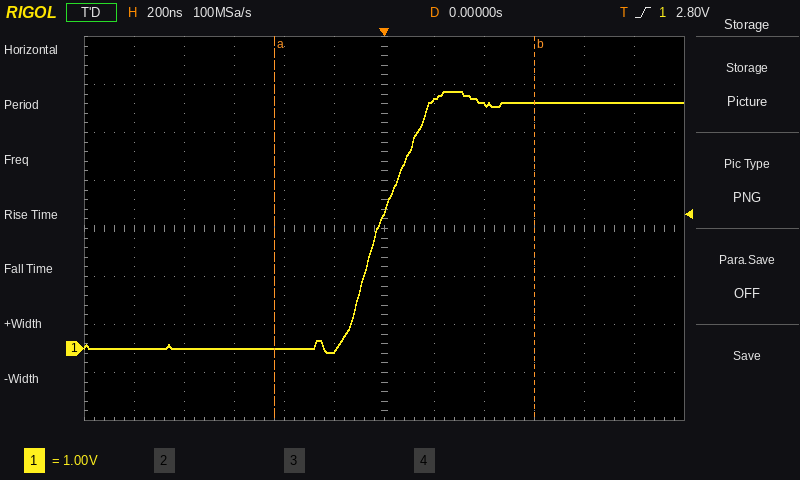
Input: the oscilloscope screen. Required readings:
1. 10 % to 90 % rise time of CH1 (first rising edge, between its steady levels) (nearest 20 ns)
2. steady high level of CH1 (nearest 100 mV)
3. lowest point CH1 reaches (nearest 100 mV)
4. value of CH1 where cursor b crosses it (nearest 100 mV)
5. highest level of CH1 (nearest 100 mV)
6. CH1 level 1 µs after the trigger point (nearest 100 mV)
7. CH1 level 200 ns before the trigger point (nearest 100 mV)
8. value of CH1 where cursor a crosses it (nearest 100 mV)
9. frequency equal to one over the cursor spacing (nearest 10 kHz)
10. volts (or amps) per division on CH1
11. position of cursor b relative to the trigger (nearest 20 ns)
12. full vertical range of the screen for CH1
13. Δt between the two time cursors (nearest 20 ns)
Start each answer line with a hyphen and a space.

- 280 ns
- 5.1 V
- -100 mV
- 5.1 V
- 5.4 V
- 5.1 V
- 0.0 V
- 0.0 V
- 960 kHz
- 1 V
- +600 ns
- 8 V
- 1.04 µs
